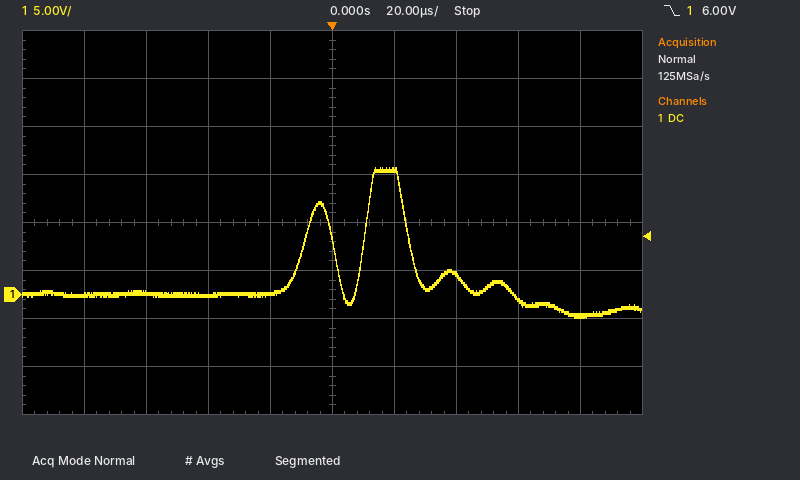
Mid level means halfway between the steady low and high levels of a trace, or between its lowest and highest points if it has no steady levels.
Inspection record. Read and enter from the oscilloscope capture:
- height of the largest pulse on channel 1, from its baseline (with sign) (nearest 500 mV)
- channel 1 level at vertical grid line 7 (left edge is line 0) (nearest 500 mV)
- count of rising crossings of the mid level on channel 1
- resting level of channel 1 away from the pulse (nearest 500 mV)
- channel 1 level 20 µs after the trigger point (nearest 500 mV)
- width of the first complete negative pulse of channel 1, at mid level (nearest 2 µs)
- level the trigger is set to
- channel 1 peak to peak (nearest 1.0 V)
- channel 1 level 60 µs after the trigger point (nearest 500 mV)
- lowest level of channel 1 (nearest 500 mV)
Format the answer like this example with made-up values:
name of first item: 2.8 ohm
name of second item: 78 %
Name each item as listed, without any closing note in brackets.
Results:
height of the largest pulse on channel 1, from its baseline (with sign): +13.0 V
channel 1 level at vertical grid line 7 (left edge is line 0): 2.0 V
count of rising crossings of the mid level on channel 1: 2
resting level of channel 1 away from the pulse: 0.0 V
channel 1 level 20 µs after the trigger point: 13.0 V
width of the first complete negative pulse of channel 1, at mid level: 10 µs
level the trigger is set to: 6.00 V
channel 1 peak to peak: 16.0 V
channel 1 level 60 µs after the trigger point: -500 mV
lowest level of channel 1: -2.5 V
